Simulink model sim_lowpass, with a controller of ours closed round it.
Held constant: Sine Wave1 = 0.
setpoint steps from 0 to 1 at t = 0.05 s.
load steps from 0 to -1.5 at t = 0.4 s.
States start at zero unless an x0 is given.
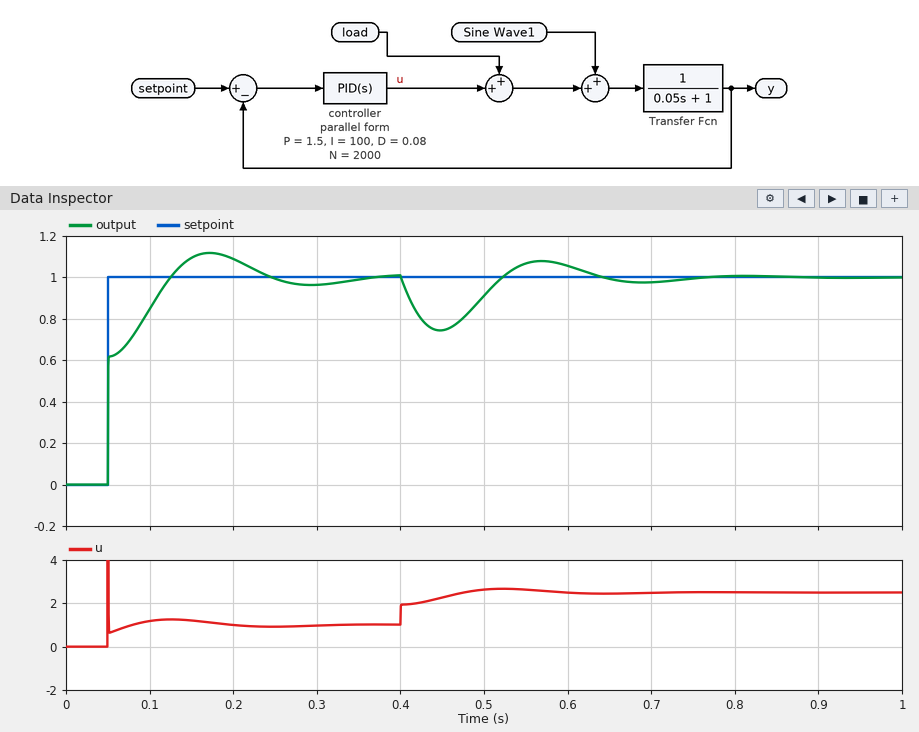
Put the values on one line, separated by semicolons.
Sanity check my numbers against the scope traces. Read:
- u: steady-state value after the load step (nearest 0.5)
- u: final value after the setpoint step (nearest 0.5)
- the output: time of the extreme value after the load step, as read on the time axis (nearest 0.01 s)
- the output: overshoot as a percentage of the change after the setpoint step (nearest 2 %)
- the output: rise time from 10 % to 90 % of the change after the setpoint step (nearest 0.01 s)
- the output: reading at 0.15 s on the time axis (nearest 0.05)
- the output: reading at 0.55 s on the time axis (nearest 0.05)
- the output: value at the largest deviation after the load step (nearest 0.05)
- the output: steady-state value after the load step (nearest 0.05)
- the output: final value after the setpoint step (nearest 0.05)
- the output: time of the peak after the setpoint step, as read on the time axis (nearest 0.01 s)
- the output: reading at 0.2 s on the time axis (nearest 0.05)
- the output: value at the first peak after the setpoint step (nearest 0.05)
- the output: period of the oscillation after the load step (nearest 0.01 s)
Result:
2.5; 1.0; 0.45 s; 12 %; 0.06 s; 1.10; 1.05; 0.75; 1.00; 1.00; 0.17 s; 1.10; 1.10; 0.24 s
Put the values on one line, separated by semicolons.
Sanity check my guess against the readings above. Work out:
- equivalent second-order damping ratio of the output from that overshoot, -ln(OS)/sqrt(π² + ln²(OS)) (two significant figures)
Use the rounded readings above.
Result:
0.56
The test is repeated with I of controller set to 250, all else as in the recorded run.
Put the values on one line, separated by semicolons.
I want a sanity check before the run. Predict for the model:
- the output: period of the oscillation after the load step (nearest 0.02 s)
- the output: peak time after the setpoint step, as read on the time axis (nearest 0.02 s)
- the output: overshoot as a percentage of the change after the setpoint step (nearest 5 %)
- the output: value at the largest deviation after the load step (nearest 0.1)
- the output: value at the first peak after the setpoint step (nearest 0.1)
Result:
0.14 s; 0.12 s; 20 %; 0.8; 1.2
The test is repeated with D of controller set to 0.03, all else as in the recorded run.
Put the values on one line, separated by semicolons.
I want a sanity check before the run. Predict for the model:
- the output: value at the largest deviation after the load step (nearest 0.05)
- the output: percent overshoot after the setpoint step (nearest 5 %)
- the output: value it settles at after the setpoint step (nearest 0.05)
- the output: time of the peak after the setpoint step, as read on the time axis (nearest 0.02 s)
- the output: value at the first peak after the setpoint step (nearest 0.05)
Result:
0.70; 15 %; 1.00; 0.14 s; 1.15
